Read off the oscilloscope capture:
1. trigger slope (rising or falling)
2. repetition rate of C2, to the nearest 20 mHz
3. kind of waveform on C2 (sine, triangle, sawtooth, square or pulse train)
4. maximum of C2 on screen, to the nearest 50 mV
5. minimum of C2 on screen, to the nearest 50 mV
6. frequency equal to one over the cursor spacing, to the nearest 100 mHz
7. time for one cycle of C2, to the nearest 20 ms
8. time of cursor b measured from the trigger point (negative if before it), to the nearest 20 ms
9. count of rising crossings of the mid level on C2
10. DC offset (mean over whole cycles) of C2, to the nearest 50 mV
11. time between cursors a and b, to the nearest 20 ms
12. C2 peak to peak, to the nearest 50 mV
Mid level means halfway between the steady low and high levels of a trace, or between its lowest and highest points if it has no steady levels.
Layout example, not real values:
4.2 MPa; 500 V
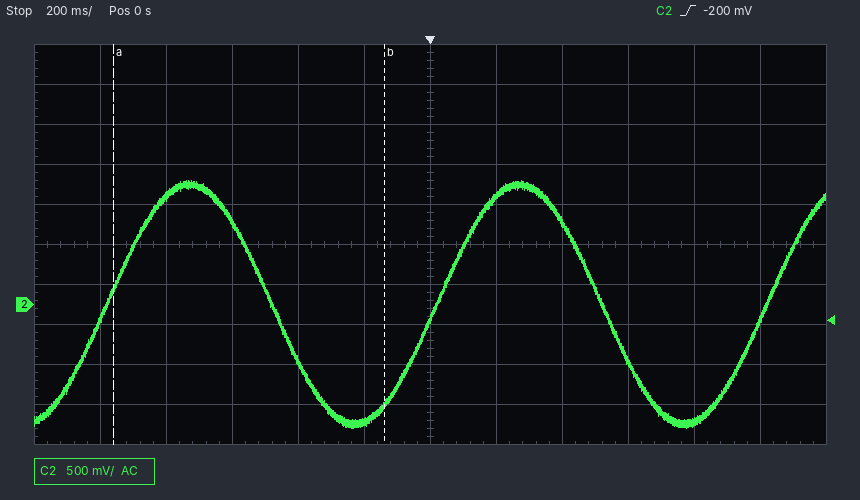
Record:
rising; 1.00 Hz; sine; 1.55 V; -1.55 V; 1.2 Hz; 1.00 s; -140 ms; 3; 0 mV; 820 ms; 3.10 V
